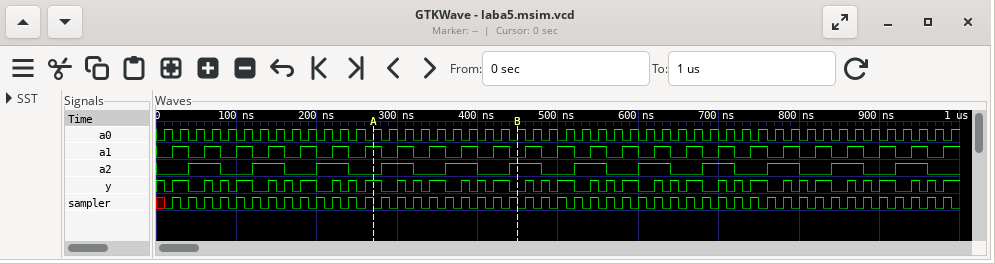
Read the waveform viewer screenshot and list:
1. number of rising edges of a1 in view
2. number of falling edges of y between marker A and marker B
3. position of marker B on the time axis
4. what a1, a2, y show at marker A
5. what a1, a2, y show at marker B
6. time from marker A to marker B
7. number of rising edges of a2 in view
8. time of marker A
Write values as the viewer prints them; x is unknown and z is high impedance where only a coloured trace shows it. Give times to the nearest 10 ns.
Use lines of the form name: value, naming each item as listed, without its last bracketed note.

number of rising edges of a1 in view: 25
number of falling edges of y between marker A and marker B: 7
position of marker B on the time axis: 450 ns
what a1, a2, y show at marker A: a1=1, a2=0, y=1
what a1, a2, y show at marker B: a1=0, a2=1, y=0
time from marker A to marker B: 180 ns
number of rising edges of a2 in view: 12
time of marker A: 270 ns
